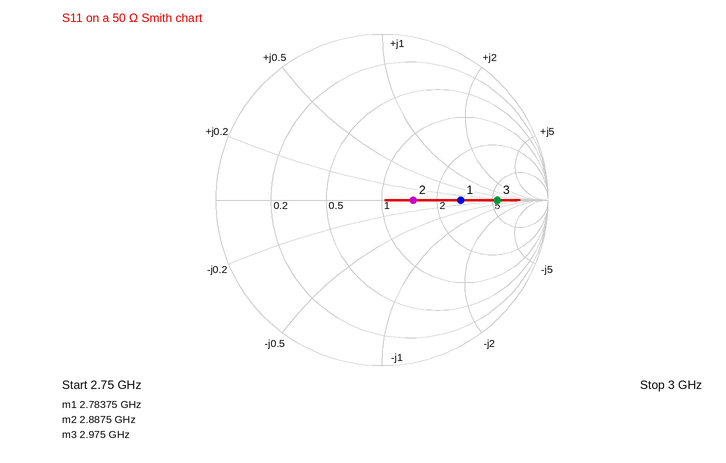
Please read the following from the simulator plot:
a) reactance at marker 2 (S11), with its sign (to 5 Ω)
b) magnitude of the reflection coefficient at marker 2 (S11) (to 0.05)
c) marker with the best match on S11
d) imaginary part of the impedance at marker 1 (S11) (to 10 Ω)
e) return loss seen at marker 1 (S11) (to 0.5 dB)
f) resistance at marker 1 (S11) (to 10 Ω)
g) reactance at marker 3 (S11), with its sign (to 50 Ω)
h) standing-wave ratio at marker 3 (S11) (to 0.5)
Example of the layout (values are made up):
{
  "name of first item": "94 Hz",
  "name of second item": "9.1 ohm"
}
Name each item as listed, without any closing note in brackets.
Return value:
{
  "reactance at marker 2 (S11), with its sign": "0 Ω",
  "magnitude of the reflection coefficient at marker 2 (S11)": "0.20",
  "marker with the best match on S11": "marker 2",
  "imaginary part of the impedance at marker 1 (S11)": "0 Ω",
  "return loss seen at marker 1 (S11)": "6.5 dB",
  "resistance at marker 1 (S11)": "140 Ω",
  "reactance at marker 3 (S11), with its sign": "0 Ω",
  "standing-wave ratio at marker 3 (S11)": "5.5"
}
